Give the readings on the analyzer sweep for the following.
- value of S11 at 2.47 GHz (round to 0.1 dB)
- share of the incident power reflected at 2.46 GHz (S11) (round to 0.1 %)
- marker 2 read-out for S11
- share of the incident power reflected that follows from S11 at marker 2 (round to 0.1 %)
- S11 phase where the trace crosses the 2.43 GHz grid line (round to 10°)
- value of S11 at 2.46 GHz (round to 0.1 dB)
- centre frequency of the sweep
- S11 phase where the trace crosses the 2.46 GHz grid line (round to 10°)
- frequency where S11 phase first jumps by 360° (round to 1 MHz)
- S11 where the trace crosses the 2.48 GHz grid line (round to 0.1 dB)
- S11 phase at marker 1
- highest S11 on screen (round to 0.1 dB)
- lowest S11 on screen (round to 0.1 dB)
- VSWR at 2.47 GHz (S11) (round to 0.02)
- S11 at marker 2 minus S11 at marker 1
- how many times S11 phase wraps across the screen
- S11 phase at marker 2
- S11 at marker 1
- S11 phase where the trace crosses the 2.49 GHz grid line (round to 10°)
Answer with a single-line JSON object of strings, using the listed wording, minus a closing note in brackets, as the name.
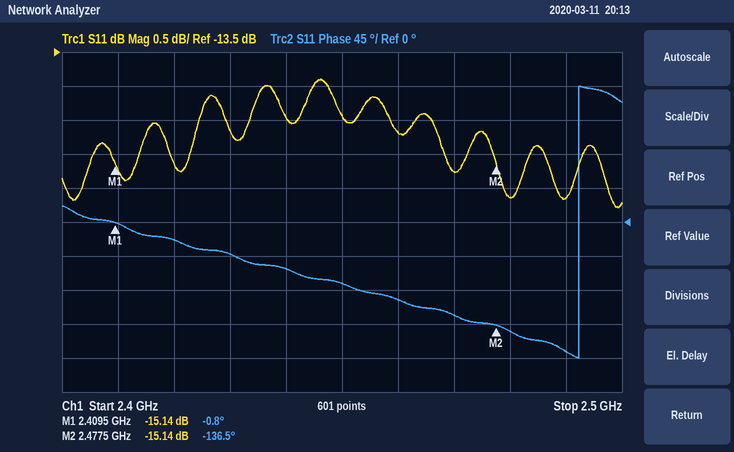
{"value of S11 at 2.47 GHz": "-15.3 dB", "share of the incident power reflected at 2.46 GHz (S11)": "3.4 %", "marker 2 read-out for S11": "-15.14 dB", "share of the incident power reflected that follows from S11 at marker 2": "3.1 %", "S11 phase where the trace crosses the 2.43 GHz grid line": "-40°", "value of S11 at 2.46 GHz": "-14.7 dB", "centre frequency of the sweep": "2.45 GHz", "S11 phase where the trace crosses the 2.46 GHz grid line": "-100°", "frequency where S11 phase first jumps by 360°": "2.492 GHz", "S11 where the trace crosses the 2.48 GHz grid line": "-15.6 dB", "S11 phase at marker 1": "-0.8°", "highest S11 on screen": "-13.9 dB", "lowest S11 on screen": "-15.8 dB", "VSWR at 2.47 GHz (S11)": "1.42", "S11 at marker 2 minus S11 at marker 1": "0.00 dB", "how many times S11 phase wraps across the screen": "1", "S11 phase at marker 2": "-136.5°", "S11 at marker 1": "-15.14 dB", "S11 phase where the trace crosses the 2.49 GHz grid line": "-170°"}
